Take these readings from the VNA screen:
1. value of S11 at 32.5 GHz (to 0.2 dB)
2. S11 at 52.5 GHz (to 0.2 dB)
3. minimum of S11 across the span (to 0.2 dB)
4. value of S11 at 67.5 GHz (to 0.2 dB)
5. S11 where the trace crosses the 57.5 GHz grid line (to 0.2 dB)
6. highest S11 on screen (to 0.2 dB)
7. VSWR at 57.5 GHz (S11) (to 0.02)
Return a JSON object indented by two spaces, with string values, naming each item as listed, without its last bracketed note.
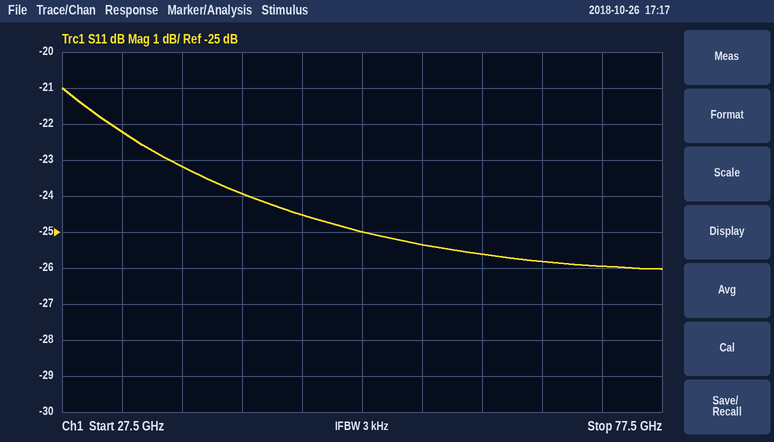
{
  "value of S11 at 32.5 GHz": "-22.2 dB",
  "S11 at 52.5 GHz": "-25.0 dB",
  "minimum of S11 across the span": "-26.0 dB",
  "value of S11 at 67.5 GHz": "-25.8 dB",
  "S11 where the trace crosses the 57.5 GHz grid line": "-25.4 dB",
  "highest S11 on screen": "-21.0 dB",
  "VSWR at 57.5 GHz (S11)": "1.12"
}
